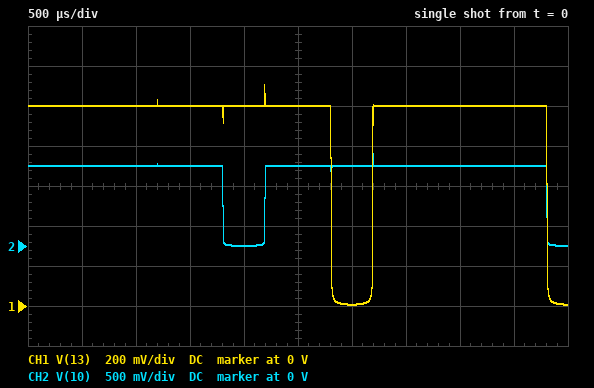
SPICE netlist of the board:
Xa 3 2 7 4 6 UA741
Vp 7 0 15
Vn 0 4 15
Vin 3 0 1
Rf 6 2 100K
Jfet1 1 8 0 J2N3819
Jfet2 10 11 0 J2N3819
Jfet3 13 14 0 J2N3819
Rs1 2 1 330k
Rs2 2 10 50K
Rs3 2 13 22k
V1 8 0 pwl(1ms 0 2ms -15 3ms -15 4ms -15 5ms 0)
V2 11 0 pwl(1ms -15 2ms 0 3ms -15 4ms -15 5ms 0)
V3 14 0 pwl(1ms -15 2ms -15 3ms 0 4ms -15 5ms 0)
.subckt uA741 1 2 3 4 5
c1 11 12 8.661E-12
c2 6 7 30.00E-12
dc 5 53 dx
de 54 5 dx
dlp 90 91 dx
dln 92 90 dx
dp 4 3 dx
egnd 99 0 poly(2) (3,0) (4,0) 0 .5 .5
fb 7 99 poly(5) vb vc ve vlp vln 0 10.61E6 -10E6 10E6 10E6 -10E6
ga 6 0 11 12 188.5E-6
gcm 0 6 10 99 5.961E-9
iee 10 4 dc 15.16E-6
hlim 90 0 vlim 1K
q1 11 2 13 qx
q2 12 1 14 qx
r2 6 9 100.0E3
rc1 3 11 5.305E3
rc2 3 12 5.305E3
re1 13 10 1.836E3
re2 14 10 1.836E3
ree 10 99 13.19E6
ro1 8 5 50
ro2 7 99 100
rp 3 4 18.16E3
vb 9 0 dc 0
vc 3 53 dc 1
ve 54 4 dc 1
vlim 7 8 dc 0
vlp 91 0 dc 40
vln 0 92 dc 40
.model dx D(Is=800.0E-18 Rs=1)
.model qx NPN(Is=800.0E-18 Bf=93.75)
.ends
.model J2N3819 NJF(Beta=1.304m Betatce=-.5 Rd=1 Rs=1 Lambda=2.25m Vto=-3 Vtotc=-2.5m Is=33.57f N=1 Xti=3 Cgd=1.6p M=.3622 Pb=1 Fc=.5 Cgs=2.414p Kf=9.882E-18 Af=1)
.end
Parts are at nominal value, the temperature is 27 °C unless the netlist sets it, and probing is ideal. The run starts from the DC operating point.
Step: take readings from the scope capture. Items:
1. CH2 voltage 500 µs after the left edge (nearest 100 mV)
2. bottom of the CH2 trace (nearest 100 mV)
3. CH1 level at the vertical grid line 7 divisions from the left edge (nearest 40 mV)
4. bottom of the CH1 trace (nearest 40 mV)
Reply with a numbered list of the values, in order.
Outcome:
1. 1.0 V
2. 0 V
3. 1.00 V
4. 0 V
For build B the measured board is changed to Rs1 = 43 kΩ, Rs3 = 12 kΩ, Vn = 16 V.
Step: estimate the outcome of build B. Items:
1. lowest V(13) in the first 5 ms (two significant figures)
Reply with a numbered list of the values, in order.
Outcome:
1. 11 mV
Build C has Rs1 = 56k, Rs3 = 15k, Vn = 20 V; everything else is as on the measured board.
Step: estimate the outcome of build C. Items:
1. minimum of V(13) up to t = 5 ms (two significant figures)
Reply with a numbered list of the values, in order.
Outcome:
1. 8.6 mV
